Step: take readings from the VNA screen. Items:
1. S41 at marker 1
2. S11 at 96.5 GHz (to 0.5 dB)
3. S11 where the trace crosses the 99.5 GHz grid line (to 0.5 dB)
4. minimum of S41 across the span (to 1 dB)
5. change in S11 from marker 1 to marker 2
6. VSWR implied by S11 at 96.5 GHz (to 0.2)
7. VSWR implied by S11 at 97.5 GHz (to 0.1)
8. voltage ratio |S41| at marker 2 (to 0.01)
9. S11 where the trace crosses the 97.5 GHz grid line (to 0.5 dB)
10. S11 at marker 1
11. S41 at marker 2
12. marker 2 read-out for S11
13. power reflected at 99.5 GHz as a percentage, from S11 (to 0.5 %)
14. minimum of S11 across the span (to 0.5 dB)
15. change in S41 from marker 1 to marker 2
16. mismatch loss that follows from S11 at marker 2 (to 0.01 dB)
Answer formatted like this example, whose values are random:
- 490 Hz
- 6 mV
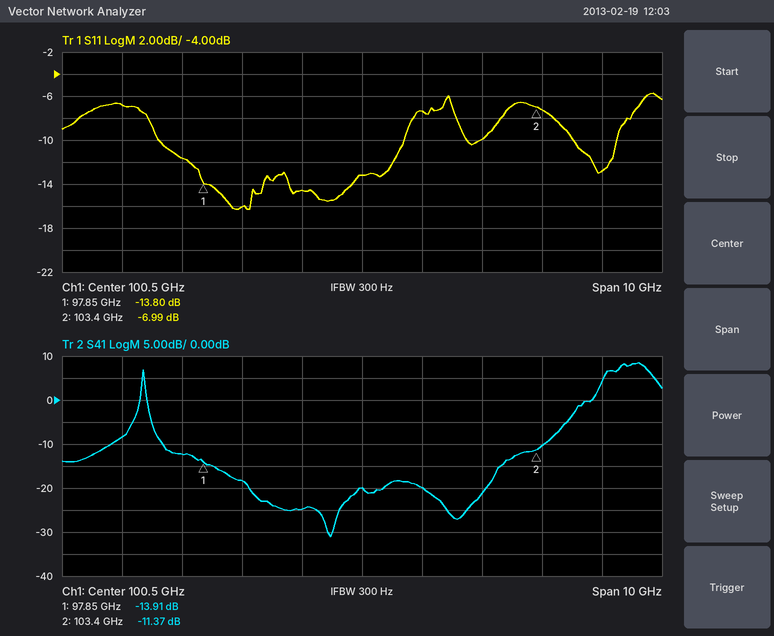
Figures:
- -13.91 dB
- -7.0 dB
- -14.5 dB
- -31 dB
- 6.81 dB
- 2.6
- 1.7
- 0.27
- -11.5 dB
- -13.80 dB
- -11.37 dB
- -6.99 dB
- 3.5 %
- -16.5 dB
- 2.54 dB
- 0.97 dB
